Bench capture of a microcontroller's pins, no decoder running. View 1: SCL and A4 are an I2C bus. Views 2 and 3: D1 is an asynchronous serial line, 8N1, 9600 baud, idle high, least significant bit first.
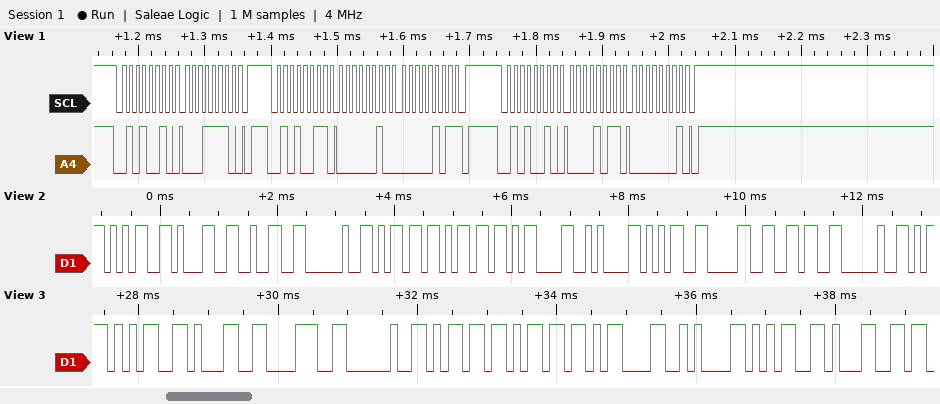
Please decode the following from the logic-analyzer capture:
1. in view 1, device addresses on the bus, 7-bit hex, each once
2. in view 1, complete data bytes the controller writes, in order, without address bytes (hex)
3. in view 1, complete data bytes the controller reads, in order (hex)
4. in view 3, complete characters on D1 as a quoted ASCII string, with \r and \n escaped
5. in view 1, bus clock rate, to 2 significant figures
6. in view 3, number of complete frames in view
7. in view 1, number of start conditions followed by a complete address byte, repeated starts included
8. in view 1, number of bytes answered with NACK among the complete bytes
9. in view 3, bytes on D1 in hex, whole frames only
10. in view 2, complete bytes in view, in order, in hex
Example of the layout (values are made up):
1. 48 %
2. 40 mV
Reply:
1. 0x29
2. 1E 0B 01
3. 02 05
4. "518 mm\r\n51"
5. 100 kHz
6. 10
7. 3
8. 1
9. 0x35 0x31 0x38 0x20 0x6D 0x6D 0x0D 0x0A 0x35 0x31
10. 0x35 0x31 0x32 0x20 0x6D 0x6D 0x0D 0x0A 0x35 0x30 0x36 0x20
